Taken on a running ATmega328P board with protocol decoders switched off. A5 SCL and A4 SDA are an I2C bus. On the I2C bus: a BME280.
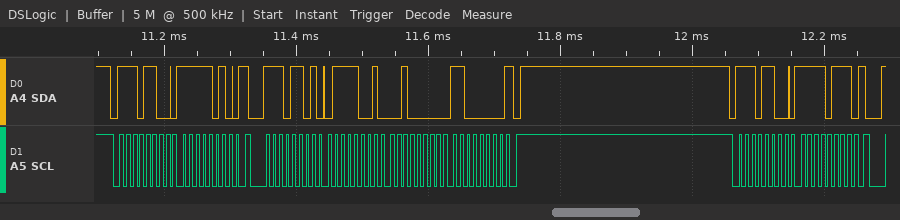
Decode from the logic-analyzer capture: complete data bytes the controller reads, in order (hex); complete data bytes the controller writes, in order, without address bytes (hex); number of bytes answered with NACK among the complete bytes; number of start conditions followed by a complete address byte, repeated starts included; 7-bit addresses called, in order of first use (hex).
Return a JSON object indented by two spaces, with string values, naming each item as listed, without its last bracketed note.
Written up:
{
  "complete data bytes the controller reads, in order": "79 20 C0",
  "complete data bytes the controller writes, in order, without address bytes": "FA F7",
  "number of bytes answered with NACK among the complete bytes": "1",
  "number of start conditions followed by a complete address byte, repeated starts included": "3",
  "7-bit addresses called, in order of first use": "0x76"
}
